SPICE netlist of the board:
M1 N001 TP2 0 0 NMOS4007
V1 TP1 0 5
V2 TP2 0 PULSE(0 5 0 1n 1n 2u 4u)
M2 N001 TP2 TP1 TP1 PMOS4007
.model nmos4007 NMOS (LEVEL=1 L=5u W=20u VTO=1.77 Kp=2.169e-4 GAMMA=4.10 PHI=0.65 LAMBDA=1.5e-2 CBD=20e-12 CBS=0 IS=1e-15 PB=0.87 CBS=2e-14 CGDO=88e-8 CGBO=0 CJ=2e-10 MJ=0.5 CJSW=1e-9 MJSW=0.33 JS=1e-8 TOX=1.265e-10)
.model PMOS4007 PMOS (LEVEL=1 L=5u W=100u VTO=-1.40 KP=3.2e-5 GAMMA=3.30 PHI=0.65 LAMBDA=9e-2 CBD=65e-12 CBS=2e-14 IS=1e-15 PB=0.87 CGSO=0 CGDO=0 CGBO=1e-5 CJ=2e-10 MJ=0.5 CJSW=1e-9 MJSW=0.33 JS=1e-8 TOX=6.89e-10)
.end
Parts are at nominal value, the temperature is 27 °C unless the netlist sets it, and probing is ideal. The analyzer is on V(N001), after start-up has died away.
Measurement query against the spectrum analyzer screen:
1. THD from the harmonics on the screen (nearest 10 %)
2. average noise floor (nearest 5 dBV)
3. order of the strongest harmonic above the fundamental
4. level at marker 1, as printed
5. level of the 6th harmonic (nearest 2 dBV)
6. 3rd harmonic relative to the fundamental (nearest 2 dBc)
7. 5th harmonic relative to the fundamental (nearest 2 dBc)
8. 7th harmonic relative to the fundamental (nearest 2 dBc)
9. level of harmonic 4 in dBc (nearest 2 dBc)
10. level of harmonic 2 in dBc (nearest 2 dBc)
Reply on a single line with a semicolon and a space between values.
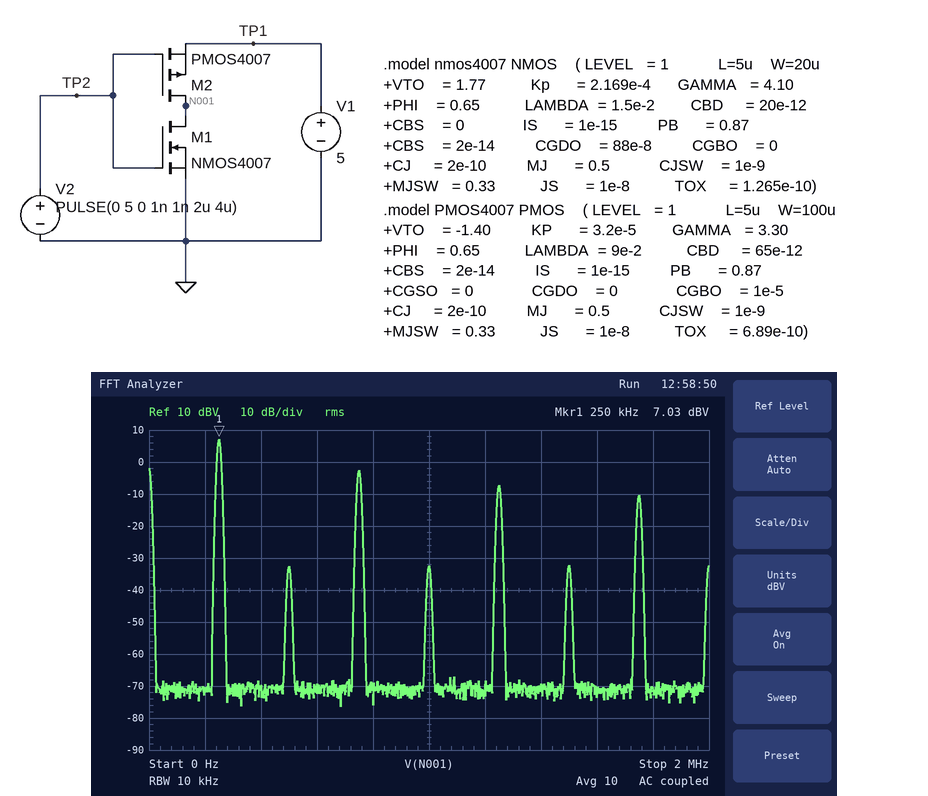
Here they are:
40 %; -70 dBV; 3; 7.03 dBV; -32 dBV; -10 dBc; -14 dBc; -18 dBc; -40 dBc; -40 dBc
